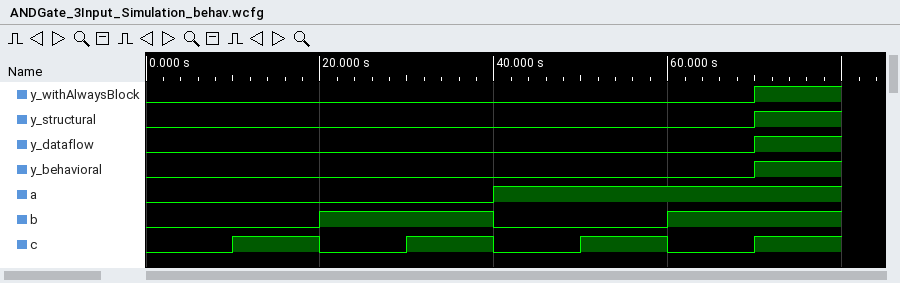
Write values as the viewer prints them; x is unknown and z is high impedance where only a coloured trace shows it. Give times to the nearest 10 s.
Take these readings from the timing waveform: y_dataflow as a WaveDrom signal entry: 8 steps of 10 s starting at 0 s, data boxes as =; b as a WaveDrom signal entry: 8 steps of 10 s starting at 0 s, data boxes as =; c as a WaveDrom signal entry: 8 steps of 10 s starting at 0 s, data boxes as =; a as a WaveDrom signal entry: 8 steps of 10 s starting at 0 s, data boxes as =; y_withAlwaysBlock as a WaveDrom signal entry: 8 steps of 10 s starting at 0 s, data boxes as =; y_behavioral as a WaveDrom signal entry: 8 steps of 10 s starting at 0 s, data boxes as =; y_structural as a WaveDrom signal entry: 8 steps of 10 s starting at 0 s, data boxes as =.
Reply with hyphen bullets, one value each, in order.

- {name: 'y_dataflow', wave: '0......1'}
- {name: 'b', wave: '0.1.0.1.'}
- {name: 'c', wave: '01010101'}
- {name: 'a', wave: '0...1...'}
- {name: 'y_withAlwaysBlock', wave: '0......1'}
- {name: 'y_behavioral', wave: '0......1'}
- {name: 'y_structural', wave: '0......1'}
